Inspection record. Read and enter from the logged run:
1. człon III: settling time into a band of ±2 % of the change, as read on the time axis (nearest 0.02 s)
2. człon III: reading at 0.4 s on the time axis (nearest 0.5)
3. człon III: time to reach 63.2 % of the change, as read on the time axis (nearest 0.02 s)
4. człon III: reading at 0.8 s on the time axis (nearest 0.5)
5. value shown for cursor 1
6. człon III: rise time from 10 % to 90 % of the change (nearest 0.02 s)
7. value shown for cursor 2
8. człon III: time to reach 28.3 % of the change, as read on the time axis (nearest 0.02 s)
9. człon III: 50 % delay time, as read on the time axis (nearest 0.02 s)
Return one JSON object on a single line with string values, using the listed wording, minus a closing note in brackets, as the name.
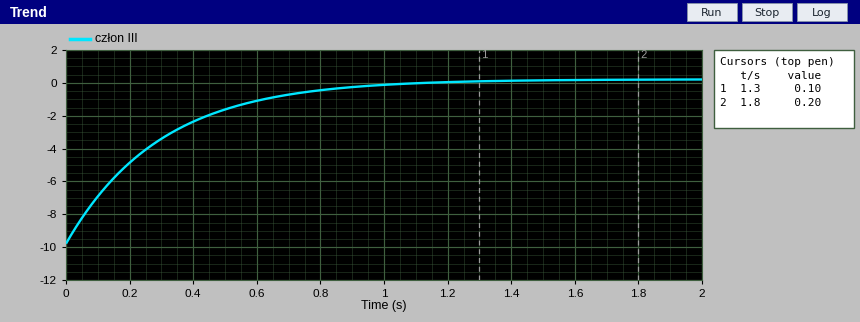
{"człon III: settling time into a band of ±2 % of the change, as read on the time axis": "1.16 s", "człon III: reading at 0.4 s on the time axis": "-2.5", "człon III: time to reach 63.2 % of the change, as read on the time axis": "0.30 s", "człon III: reading at 0.8 s on the time axis": "-0.5", "value shown for cursor 1": "0.10", "człon III: rise time from 10 % to 90 % of the change": "0.64 s", "value shown for cursor 2": "0.20", "człon III: time to reach 28.3 % of the change, as read on the time axis": "0.10 s", "człon III: 50 % delay time, as read on the time axis": "0.20 s"}
